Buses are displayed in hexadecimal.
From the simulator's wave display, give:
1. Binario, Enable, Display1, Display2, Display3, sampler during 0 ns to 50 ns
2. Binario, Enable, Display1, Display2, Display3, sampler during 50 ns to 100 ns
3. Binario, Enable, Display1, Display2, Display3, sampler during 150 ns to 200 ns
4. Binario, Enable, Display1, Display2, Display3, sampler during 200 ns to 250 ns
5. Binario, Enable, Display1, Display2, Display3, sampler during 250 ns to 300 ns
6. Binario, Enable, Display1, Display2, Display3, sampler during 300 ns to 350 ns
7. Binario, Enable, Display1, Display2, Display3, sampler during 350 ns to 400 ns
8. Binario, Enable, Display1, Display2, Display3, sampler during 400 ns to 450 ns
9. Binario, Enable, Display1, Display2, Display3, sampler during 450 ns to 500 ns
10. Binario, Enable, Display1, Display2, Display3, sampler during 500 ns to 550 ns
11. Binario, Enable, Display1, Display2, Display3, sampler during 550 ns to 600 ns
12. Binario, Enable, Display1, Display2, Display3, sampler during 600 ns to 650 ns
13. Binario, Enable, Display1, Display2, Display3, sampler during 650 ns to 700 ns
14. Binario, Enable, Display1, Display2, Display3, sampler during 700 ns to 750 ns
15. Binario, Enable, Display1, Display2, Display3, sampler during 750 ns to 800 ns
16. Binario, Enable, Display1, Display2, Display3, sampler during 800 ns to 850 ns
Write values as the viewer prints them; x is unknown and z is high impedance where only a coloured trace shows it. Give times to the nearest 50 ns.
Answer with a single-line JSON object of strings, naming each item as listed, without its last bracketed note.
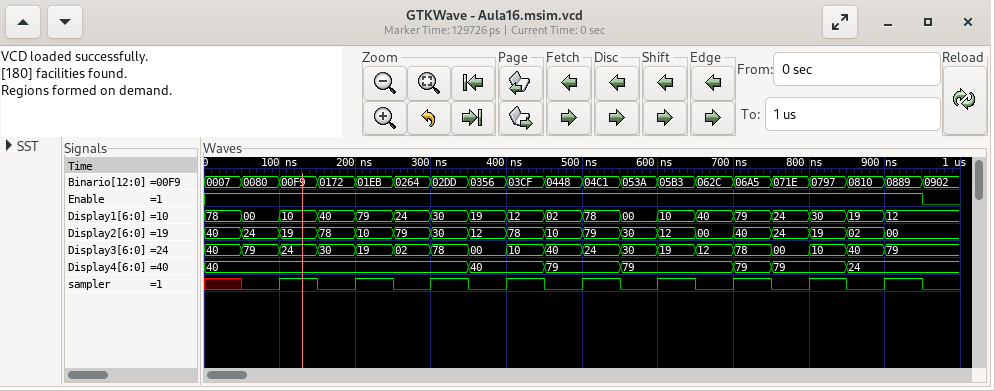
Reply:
{"Binario, Enable, Display1, Display2, Display3, sampler during 0 ns to 50 ns": "Binario=0007, Enable=1, Display1=78, Display2=40, Display3=40, sampler=x", "Binario, Enable, Display1, Display2, Display3, sampler during 50 ns to 100 ns": "Binario=0080, Enable=1, Display1=00, Display2=24, Display3=79, sampler=0", "Binario, Enable, Display1, Display2, Display3, sampler during 150 ns to 200 ns": "Binario=0172, Enable=1, Display1=40, Display2=78, Display3=30, sampler=0", "Binario, Enable, Display1, Display2, Display3, sampler during 200 ns to 250 ns": "Binario=01EB, Enable=1, Display1=79, Display2=10, Display3=19, sampler=1", "Binario, Enable, Display1, Display2, Display3, sampler during 250 ns to 300 ns": "Binario=0264, Enable=1, Display1=24, Display2=79, Display3=02, sampler=0", "Binario, Enable, Display1, Display2, Display3, sampler during 300 ns to 350 ns": "Binario=02DD, Enable=1, Display1=30, Display2=30, Display3=78, sampler=1", "Binario, Enable, Display1, Display2, Display3, sampler during 350 ns to 400 ns": "Binario=0356, Enable=1, Display1=19, Display2=12, Display3=00, sampler=0", "Binario, Enable, Display1, Display2, Display3, sampler during 400 ns to 450 ns": "Binario=03CF, Enable=1, Display1=12, Display2=78, Display3=10, sampler=1", "Binario, Enable, Display1, Display2, Display3, sampler during 450 ns to 500 ns": "Binario=0448, Enable=1, Display1=02, Display2=10, Display3=40, sampler=0", "Binario, Enable, Display1, Display2, Display3, sampler during 500 ns to 550 ns": "Binario=04C1, Enable=1, Display1=78, Display2=79, Display3=24, sampler=1", "Binario, Enable, Display1, Display2, Display3, sampler during 550 ns to 600 ns": "Binario=053A, Enable=1, Display1=00, Display2=30, Display3=30, sampler=0", "Binario, Enable, Display1, Display2, Display3, sampler during 600 ns to 650 ns": "Binario=05B3, Enable=1, Display1=10, Display2=12, Display3=19, sampler=1", "Binario, Enable, Display1, Display2, Display3, sampler during 650 ns to 700 ns": "Binario=062C, Enable=1, Display1=40, Display2=00, Display3=12, sampler=0", "Binario, Enable, Display1, Display2, Display3, sampler during 700 ns to 750 ns": "Binario=06A5, Enable=1, Display1=79, Display2=40, Display3=78, sampler=1", "Binario, Enable, Display1, Display2, Display3, sampler during 750 ns to 800 ns": "Binario=071E, Enable=1, Display1=24, Display2=24, Display3=00, sampler=0", "Binario, Enable, Display1, Display2, Display3, sampler during 800 ns to 850 ns": "Binario=0797, Enable=1, Display1=30, Display2=19, Display3=10, sampler=1"}
